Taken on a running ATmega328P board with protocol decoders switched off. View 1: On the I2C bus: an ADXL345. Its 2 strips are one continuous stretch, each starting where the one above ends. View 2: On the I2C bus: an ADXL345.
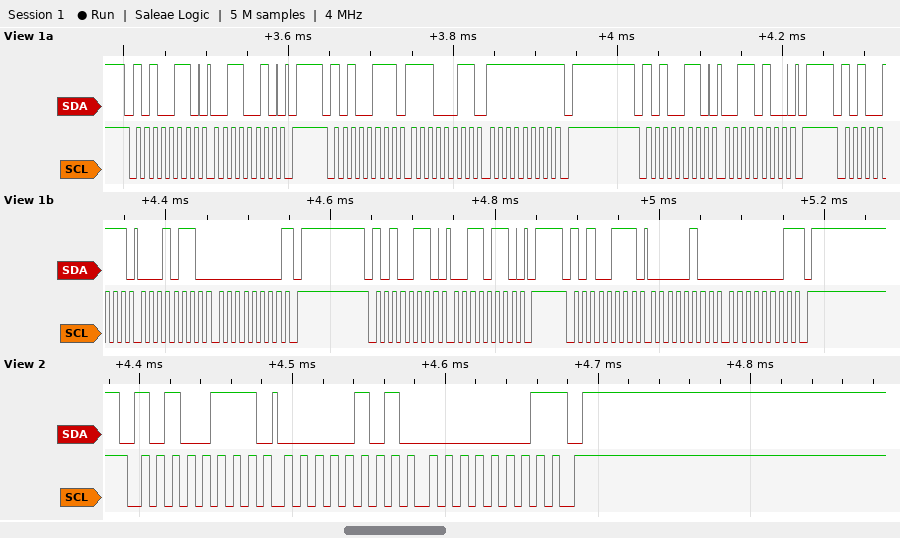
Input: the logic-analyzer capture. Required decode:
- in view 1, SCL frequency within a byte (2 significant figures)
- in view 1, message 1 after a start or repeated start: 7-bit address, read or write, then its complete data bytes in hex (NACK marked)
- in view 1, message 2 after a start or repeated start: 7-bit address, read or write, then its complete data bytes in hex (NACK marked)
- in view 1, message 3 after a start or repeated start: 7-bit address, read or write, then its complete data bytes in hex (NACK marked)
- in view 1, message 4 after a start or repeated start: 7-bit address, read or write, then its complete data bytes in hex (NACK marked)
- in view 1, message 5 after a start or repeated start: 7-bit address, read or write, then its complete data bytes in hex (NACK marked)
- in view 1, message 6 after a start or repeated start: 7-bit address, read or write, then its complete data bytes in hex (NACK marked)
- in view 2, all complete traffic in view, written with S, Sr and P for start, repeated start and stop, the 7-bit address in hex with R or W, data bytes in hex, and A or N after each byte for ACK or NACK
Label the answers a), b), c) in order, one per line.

a) 100 kHz
b) 0x53 write: 32
c) 0x53 read: E3 FF NACK
d) 0x53 write: 34
e) 0x53 read: 16 00 NACK
f) 0x53 write: 36
g) 0x53 read: 04 01 NACK
h) S 53R A 05 A 01 N P
